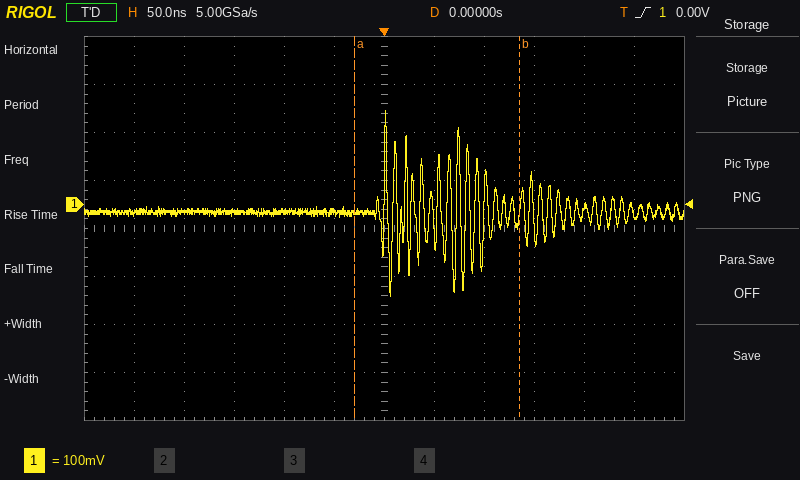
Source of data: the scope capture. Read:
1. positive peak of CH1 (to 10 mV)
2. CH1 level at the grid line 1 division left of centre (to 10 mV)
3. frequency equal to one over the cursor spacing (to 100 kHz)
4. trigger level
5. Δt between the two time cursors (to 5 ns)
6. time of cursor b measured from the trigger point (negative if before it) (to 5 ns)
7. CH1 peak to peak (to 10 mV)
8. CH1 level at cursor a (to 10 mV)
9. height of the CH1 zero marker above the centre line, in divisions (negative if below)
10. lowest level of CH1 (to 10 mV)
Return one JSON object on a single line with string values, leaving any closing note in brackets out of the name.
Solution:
{"positive peak of CH1": "200 mV", "CH1 level at the grid line 1 division left of centre": "-20 mV", "frequency equal to one over the cursor spacing": "6.1 MHz", "trigger level": "0.00 V", "Δt between the two time cursors": "165 ns", "time of cursor b measured from the trigger point (negative if before it)": "+135 ns", "CH1 peak to peak": "390 mV", "CH1 level at cursor a": "-20 mV", "height of the CH1 zero marker above the centre line, in divisions": "+0.5 div", "lowest level of CH1": "-190 mV"}
